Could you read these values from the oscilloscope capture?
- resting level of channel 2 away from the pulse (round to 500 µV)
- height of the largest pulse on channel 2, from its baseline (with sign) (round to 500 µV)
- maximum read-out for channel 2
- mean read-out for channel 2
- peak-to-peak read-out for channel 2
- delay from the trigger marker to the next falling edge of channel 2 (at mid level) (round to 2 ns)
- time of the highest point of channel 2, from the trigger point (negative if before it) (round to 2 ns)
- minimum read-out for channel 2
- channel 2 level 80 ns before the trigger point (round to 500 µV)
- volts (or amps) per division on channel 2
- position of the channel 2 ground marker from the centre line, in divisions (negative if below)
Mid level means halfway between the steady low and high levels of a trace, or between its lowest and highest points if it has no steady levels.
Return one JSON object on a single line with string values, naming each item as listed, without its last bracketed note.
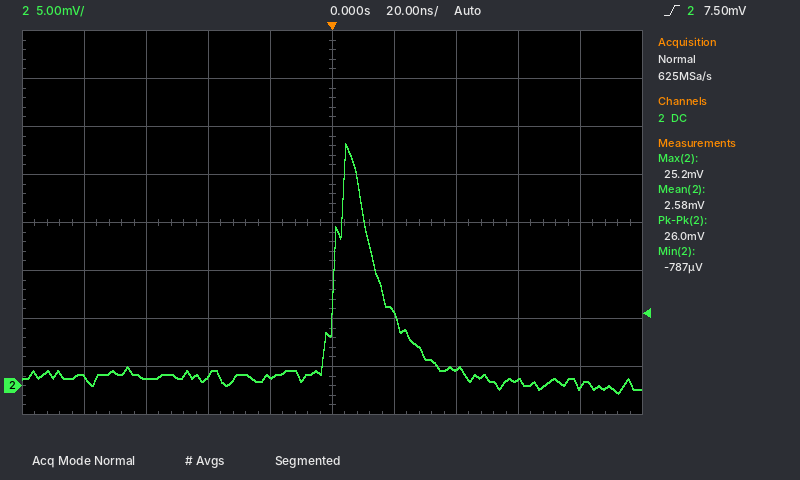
{"resting level of channel 2 away from the pulse": "1.0 mV", "height of the largest pulse on channel 2, from its baseline (with sign)": "+24.0 mV", "maximum read-out for channel 2": "25.2 mV", "mean read-out for channel 2": "2.58 mV", "peak-to-peak read-out for channel 2": "26.0 mV", "delay from the trigger marker to the next falling edge of channel 2 (at mid level)": "14 ns", "time of the highest point of channel 2, from the trigger point (negative if before it)": "+4 ns", "minimum read-out for channel 2": "-787 µV", "channel 2 level 80 ns before the trigger point": "1.0 mV", "volts (or amps) per division on channel 2": "5 mV", "position of the channel 2 ground marker from the centre line, in divisions": "-3.4 div"}
